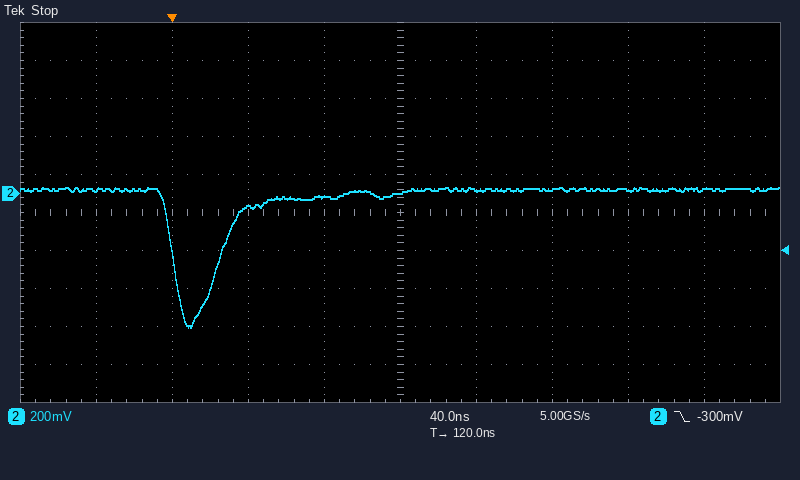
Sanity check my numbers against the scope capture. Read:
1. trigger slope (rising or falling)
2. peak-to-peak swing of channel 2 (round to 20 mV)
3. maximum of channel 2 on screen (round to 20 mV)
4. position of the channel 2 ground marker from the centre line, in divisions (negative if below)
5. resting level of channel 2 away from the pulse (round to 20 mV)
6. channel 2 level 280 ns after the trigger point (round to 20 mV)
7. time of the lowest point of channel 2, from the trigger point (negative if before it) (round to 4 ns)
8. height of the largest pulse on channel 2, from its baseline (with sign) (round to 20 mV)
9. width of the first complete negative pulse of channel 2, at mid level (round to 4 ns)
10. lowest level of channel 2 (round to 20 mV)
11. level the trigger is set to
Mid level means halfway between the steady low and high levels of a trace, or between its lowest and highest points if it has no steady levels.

falling
740 mV
40 mV
+0.5 div
20 mV
20 mV
+8 ns
-720 mV
24 ns
-700 mV
-300 mV
